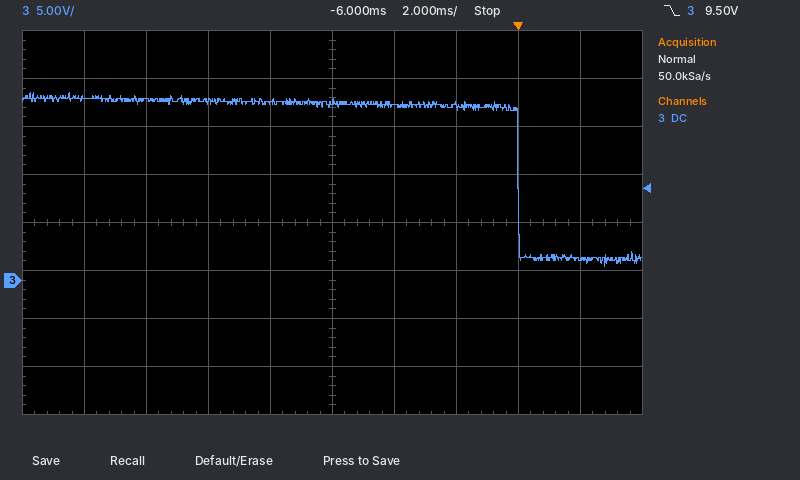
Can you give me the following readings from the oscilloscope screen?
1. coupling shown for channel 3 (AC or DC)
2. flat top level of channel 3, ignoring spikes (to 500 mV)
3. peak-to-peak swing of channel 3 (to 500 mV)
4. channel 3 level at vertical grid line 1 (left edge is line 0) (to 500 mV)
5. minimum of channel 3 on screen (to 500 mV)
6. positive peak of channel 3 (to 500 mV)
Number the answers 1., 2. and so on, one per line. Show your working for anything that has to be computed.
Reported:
1. DC
2. 18.5 V
3. 19.5 V − (1.5 V) = 18.0 V
4. 19.0 V
5. 1.5 V
6. 19.5 V
